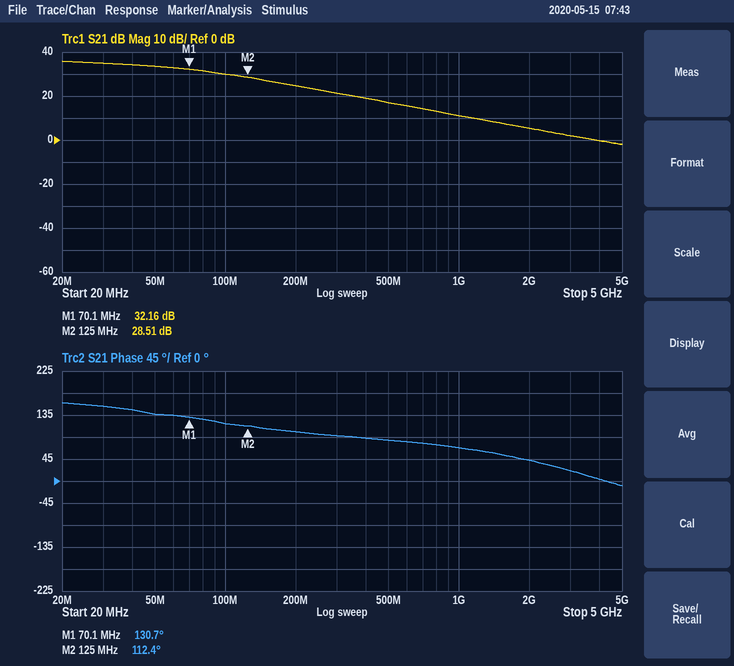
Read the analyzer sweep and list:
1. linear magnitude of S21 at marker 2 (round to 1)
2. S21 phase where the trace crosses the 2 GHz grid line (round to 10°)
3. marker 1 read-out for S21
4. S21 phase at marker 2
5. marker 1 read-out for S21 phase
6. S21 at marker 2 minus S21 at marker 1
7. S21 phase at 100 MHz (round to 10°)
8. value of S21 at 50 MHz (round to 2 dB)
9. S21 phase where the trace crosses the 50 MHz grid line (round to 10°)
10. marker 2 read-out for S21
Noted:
27
40°
32.16 dB
112.4°
130.7°
-3.65 dB
120°
34 dB
140°
28.51 dB
